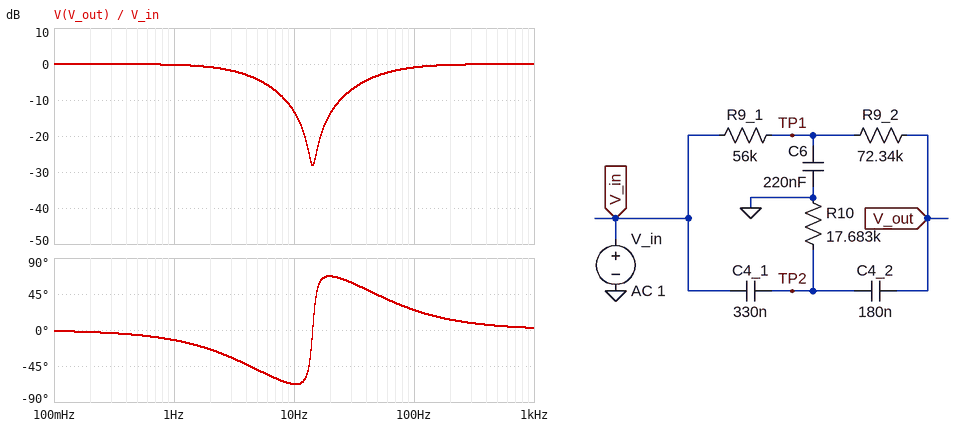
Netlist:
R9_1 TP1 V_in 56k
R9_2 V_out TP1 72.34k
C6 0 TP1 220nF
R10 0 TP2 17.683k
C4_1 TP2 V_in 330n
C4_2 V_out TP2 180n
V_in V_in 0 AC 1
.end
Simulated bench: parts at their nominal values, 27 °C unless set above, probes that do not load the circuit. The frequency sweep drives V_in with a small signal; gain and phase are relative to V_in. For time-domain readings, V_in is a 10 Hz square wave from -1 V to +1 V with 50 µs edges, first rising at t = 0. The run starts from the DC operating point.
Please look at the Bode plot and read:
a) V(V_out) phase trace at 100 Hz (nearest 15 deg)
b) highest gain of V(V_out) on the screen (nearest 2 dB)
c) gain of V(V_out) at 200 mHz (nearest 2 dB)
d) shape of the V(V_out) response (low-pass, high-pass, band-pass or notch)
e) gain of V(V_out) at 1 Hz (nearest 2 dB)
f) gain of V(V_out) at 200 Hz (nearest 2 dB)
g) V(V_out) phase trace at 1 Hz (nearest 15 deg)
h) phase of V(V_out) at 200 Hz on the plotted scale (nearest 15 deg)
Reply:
30 deg
0 dB
0 dB
notch
0 dB
0 dB
-15 deg
15 deg
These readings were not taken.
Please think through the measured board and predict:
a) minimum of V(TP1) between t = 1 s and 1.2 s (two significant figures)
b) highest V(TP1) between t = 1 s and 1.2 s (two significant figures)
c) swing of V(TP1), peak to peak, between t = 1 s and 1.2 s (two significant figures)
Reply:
-760 mV
760 mV
1.5 V
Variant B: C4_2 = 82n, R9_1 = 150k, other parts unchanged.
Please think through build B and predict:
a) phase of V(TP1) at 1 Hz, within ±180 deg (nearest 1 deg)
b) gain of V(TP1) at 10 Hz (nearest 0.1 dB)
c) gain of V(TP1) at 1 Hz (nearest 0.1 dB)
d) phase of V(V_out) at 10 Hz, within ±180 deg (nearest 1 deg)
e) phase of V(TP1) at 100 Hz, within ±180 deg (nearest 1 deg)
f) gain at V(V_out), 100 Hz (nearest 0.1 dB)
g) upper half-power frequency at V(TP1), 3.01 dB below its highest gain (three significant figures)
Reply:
-16 deg
-11.0 dB
-0.4 dB
-92 deg
-61 deg
-1.3 dB
3.20 Hz
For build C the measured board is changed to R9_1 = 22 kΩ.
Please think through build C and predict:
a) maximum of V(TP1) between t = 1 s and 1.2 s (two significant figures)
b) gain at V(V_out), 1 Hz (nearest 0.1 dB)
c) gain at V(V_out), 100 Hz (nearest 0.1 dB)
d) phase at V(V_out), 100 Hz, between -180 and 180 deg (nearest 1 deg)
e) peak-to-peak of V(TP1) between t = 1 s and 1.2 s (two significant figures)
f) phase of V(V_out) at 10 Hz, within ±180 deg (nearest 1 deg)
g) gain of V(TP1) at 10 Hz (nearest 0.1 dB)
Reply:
940 mV
-0.1 dB
-1.2 dB
24 deg
1.9 V
-46 deg
-1.8 dB
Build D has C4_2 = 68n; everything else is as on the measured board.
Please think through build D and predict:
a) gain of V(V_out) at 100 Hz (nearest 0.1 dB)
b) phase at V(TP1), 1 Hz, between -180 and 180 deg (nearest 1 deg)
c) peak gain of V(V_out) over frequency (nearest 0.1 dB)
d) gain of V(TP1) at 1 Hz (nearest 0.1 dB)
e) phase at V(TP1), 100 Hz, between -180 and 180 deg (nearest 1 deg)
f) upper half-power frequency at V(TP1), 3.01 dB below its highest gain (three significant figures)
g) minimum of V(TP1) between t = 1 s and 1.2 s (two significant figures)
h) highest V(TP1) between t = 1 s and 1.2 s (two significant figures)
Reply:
-1.7 dB
-6 deg
0 dB
-0.1 dB
-64 deg
8.49 Hz
-880 mV
880 mV
